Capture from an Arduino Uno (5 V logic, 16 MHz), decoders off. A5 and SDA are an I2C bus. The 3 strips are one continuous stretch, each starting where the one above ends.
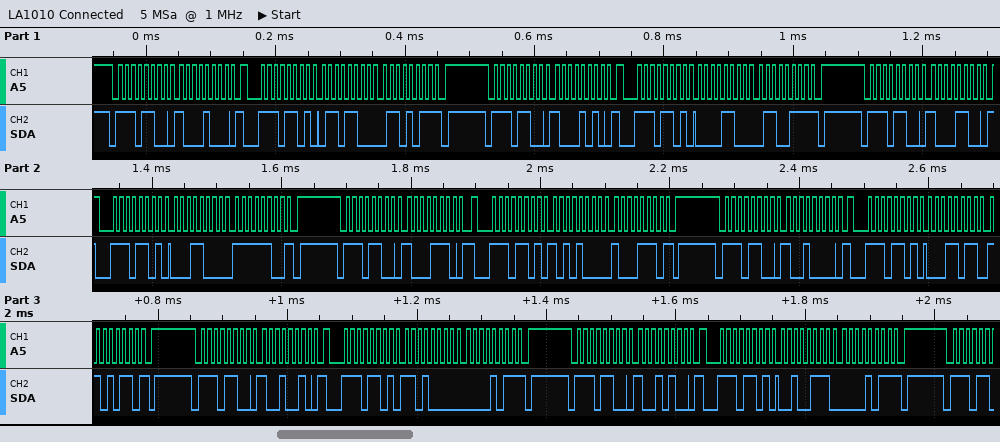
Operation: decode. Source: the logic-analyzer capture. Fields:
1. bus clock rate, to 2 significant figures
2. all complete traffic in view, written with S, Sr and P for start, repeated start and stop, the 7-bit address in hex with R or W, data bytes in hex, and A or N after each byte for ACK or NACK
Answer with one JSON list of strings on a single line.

["100 kHz", "S 76W A 88 A Sr 76R A 6C A 6B N P S 76W A 8A A Sr 76R A 0C A 67 N P S 76W A 8C A Sr 76R A 18 A FC N P S 76W A 8E A Sr 76R A A8 A 8E N P S 76W A 90 A Sr 76R A 1B A D6 N P S 76W A 92 A Sr 76R A D0 A 0B N P S 76W A 94 A Sr 76R A 27 A 0B N P"]
